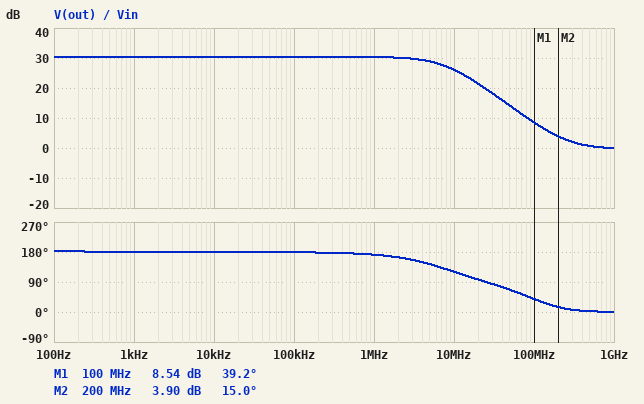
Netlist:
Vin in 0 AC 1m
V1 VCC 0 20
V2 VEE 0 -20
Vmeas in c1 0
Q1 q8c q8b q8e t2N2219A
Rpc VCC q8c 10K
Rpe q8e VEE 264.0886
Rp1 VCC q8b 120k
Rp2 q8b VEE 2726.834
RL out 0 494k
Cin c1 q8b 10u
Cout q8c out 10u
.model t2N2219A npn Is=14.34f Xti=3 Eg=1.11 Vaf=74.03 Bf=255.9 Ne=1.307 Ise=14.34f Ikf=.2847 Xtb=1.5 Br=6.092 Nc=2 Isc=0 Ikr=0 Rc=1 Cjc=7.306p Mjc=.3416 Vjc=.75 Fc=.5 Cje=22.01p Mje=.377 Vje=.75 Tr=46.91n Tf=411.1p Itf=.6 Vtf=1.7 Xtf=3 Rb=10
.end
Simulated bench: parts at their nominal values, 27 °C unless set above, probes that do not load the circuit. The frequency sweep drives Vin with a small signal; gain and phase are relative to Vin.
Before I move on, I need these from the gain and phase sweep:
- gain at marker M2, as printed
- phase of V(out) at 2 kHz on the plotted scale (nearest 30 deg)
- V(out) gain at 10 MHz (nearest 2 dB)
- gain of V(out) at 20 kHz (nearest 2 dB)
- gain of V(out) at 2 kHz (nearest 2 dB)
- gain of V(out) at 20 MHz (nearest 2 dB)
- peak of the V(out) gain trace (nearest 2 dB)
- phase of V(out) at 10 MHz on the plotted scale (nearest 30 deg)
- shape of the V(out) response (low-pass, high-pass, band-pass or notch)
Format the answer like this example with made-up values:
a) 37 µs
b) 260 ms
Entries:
a) 3.90 dB
b) 180 deg
c) 26 dB
d) 30 dB
e) 30 dB
f) 22 dB
g) 30 dB
h) 120 deg
i) low-pass
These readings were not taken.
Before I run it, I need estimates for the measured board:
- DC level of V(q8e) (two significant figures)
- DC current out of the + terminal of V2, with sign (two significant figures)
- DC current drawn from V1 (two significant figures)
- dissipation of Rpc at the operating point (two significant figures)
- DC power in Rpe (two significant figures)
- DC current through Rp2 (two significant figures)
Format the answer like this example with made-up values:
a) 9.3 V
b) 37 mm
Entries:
a) -20 V
b) -1.2 mA
c) 1.2 mA
d) 8.3 mW
e) 220 µW
f) 320 µA
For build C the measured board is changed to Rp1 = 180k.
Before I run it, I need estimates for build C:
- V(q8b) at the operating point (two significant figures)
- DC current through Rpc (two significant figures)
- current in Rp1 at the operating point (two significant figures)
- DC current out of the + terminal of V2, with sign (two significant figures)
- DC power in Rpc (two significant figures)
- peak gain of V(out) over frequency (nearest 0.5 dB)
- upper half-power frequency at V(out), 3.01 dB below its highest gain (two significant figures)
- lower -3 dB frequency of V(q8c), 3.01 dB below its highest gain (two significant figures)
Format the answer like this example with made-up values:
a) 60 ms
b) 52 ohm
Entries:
a) -19 V
b) 88 µA
c) 220 µA
d) -310 µA
e) 77 µW
f) 25.0 dB
g) 8.1 MHz
h) 6.1 Hz
